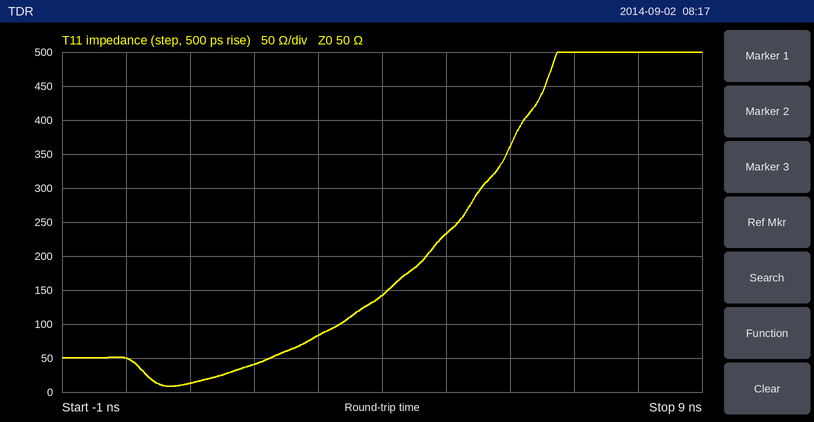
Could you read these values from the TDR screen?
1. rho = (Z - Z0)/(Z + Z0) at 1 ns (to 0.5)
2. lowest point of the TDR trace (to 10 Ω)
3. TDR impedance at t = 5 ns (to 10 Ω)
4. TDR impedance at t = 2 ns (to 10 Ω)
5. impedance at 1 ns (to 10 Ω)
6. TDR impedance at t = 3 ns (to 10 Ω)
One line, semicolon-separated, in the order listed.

-0.5; 10 Ω; 230 Ω; 40 Ω; 10 Ω; 80 Ω
